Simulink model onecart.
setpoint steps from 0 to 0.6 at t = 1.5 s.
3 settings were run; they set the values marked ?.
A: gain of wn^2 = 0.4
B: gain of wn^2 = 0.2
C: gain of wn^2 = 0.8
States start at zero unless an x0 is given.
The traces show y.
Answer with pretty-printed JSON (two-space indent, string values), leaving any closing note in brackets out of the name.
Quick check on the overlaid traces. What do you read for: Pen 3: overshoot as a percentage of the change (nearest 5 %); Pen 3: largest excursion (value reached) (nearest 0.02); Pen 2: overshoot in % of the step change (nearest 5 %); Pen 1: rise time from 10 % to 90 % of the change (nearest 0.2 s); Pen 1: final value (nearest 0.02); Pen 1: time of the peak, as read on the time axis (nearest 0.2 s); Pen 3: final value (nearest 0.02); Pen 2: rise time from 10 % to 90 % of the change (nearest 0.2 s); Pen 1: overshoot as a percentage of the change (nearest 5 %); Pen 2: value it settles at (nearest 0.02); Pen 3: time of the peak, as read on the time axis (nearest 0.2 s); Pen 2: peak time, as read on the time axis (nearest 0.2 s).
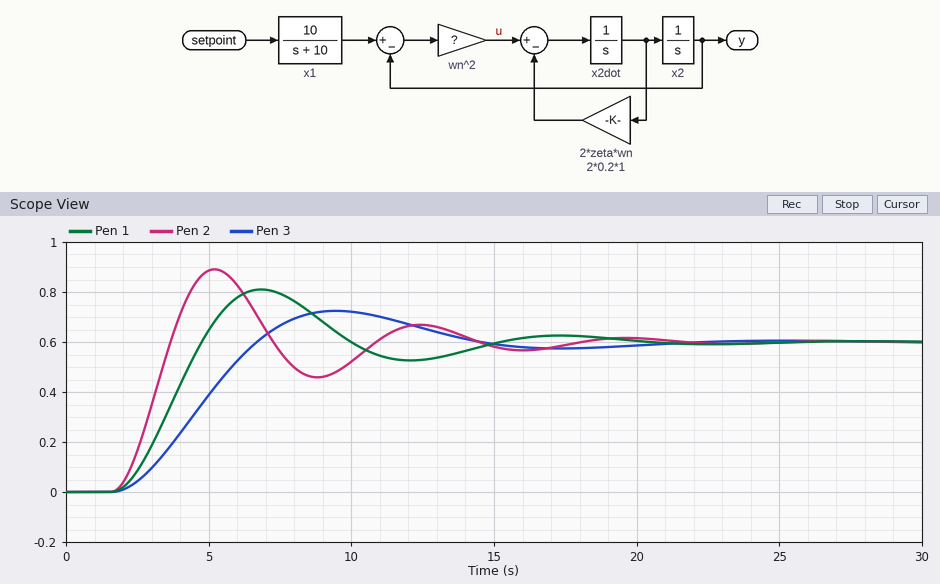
{
  "Pen 3: overshoot as a percentage of the change": "20 %",
  "Pen 3: largest excursion (value reached)": "0.72",
  "Pen 2: overshoot in % of the step change": "50 %",
  "Pen 1: rise time from 10 % to 90 % of the change": "2.2 s",
  "Pen 1: final value": "0.60",
  "Pen 1: time of the peak, as read on the time axis": "6.8 s",
  "Pen 3: final value": "0.60",
  "Pen 2: rise time from 10 % to 90 % of the change": "1.4 s",
  "Pen 1: overshoot as a percentage of the change": "35 %",
  "Pen 2: value it settles at": "0.60",
  "Pen 3: time of the peak, as read on the time axis": "9.4 s",
  "Pen 2: peak time, as read on the time axis": "5.2 s"
}
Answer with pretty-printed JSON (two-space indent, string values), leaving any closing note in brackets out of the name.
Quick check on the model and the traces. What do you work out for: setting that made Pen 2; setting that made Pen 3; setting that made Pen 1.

{
  "setting that made Pen 2": "C",
  "setting that made Pen 3": "B",
  "setting that made Pen 1": "A"
}
